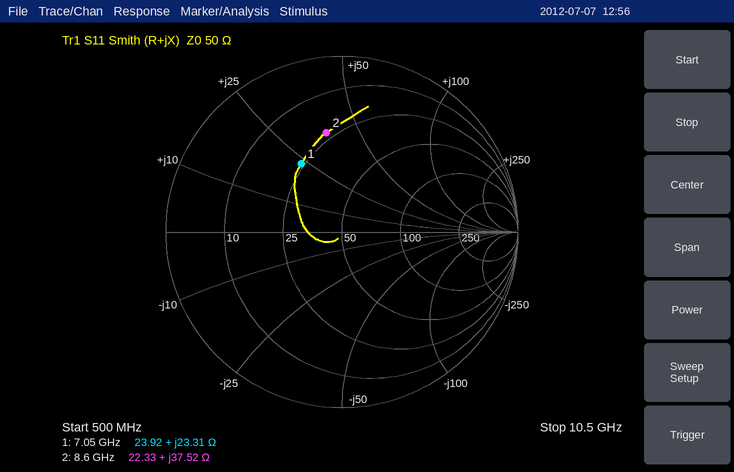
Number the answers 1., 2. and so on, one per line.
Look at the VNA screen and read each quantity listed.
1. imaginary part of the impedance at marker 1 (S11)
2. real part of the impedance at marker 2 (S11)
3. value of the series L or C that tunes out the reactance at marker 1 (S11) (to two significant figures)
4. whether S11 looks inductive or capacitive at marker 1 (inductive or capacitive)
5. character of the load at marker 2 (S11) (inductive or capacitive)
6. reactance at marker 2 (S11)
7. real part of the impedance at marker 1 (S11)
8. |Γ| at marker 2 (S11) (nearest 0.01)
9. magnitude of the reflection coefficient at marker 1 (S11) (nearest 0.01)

1. +23.31 Ω
2. 22.33 Ω
3. 970 fF
4. inductive
5. inductive
6. +37.52 Ω
7. 23.92 Ω
8. 0.57
9. 0.45
